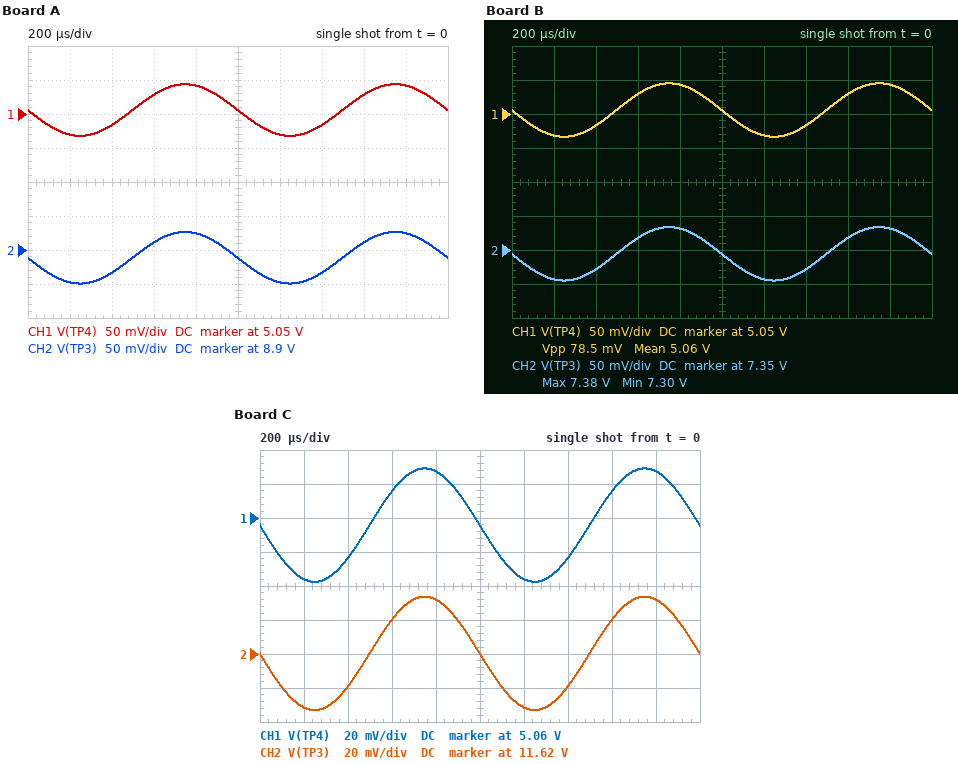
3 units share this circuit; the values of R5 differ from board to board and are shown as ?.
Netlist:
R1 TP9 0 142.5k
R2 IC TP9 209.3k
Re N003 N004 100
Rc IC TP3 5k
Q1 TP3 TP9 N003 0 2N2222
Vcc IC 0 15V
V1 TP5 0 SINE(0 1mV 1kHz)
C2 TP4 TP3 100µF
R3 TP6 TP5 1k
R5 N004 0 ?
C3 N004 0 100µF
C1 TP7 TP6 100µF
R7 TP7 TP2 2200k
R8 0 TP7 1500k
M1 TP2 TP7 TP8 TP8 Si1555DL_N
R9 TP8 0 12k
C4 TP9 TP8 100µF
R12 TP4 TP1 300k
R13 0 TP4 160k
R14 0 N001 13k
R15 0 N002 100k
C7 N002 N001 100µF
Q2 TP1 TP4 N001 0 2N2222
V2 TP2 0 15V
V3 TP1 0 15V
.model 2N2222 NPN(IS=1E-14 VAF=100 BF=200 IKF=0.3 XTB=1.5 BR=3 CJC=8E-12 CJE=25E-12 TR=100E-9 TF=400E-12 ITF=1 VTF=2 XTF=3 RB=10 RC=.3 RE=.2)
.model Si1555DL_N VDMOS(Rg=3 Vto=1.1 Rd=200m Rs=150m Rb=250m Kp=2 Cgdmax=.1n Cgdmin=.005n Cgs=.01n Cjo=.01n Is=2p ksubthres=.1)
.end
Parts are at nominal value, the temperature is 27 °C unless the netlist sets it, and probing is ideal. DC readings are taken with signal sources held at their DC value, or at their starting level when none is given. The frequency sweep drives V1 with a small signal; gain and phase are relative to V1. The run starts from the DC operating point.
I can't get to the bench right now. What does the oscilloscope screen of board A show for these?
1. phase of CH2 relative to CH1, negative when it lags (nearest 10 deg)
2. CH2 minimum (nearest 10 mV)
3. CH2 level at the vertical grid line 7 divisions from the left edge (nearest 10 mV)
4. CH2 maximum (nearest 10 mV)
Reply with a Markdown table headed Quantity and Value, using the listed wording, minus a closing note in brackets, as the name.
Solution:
| Quantity | Value |
|---|---|
| phase of CH2 relative to CH1, negative when it lags | 0 deg |
| CH2 minimum | 8.85 V |
| CH2 level at the vertical grid line 7 divisions from the left edge | 8.87 V |
| CH2 maximum | 8.93 V |
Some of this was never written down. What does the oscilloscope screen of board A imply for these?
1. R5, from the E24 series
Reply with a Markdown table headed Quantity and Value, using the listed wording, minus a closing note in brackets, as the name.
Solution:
| Quantity | Value |
|---|---|
| R5, from the E24 series | 3.9 kΩ |
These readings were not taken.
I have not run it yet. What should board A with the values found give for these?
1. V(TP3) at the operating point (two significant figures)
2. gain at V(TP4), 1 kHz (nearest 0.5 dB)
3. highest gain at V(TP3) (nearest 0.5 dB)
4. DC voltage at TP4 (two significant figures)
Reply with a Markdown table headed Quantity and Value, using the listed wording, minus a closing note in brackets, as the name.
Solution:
| Quantity | Value |
|---|---|
| V(TP3) at the operating point | 8.9 V |
| gain at V(TP4), 1 kHz | 31.5 dB |
| highest gain at V(TP3) | 31.5 dB |
| DC voltage at TP4 | 5.1 V |
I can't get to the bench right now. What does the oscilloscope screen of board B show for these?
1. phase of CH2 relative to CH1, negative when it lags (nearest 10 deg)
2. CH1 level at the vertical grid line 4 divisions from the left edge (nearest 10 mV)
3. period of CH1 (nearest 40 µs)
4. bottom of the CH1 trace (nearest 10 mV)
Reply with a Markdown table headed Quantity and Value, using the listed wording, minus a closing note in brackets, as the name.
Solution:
| Quantity | Value |
|---|---|
| phase of CH2 relative to CH1, negative when it lags | 0 deg |
| CH1 level at the vertical grid line 4 divisions from the left edge | 5.09 V |
| period of CH1 | 1.00 ms |
| bottom of the CH1 trace | 5.02 V |
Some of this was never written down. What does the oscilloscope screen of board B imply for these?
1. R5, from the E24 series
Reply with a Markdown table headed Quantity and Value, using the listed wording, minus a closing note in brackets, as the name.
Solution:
| Quantity | Value |
|---|---|
| R5, from the E24 series | 3 kΩ |
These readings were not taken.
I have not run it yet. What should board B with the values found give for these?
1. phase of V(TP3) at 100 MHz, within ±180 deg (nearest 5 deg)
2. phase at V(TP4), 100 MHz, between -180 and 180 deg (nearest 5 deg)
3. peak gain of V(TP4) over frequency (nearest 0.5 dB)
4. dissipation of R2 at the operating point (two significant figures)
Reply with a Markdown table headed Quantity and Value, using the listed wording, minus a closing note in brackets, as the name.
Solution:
| Quantity | Value |
|---|---|
| phase of V(TP3) at 100 MHz, within ±180 deg | -40 deg |
| phase at V(TP4), 100 MHz, between -180 and 180 deg | -40 deg |
| peak gain of V(TP4) over frequency | 32.0 dB |
| dissipation of R2 at the operating point | 440 µW |
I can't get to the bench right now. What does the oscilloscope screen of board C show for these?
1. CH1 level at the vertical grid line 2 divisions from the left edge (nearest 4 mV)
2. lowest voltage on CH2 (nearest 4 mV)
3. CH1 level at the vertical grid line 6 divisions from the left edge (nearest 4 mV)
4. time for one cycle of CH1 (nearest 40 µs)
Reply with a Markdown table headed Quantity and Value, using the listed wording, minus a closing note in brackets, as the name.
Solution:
| Quantity | Value |
|---|---|
| CH1 level at the vertical grid line 2 divisions from the left edge | 5.036 V |
| lowest voltage on CH2 | 11.588 V |
| CH1 level at the vertical grid line 6 divisions from the left edge | 5.024 V |
| time for one cycle of CH1 | 1.00 ms |
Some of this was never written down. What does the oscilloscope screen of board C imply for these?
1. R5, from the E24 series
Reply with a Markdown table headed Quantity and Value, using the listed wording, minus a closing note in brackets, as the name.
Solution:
| Quantity | Value |
|---|---|
| R5, from the E24 series | 7.5 kΩ |
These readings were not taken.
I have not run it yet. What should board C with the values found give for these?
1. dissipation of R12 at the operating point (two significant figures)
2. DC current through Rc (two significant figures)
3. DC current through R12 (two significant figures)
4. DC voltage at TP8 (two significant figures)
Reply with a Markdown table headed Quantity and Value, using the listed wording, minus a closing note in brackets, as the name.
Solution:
| Quantity | Value |
|---|---|
| dissipation of R12 at the operating point | 330 µW |
| DC current through Rc | 680 µA |
| DC current through R12 | 33 µA |
| DC voltage at TP8 | 5.1 V |
